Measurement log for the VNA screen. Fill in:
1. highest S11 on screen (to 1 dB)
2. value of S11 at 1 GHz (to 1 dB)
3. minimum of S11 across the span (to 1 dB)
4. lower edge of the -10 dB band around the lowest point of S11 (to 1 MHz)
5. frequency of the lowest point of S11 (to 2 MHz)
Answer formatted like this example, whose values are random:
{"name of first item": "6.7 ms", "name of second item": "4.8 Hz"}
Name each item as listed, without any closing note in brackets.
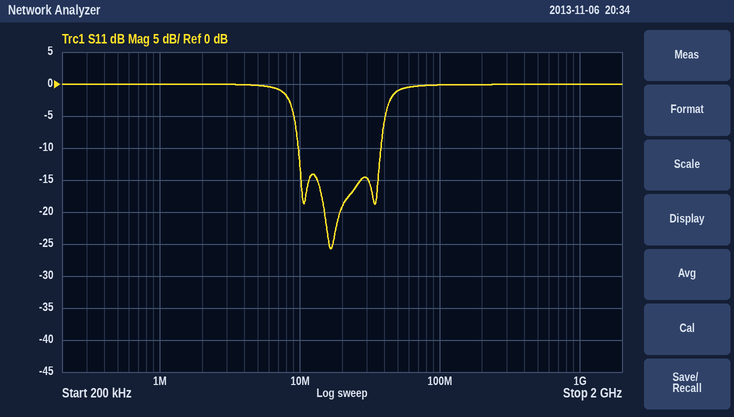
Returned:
{"highest S11 on screen": "0 dB", "value of S11 at 1 GHz": "0 dB", "minimum of S11 across the span": "-26 dB", "lower edge of the -10 dB band around the lowest point of S11": "10 MHz", "frequency of the lowest point of S11": "16 MHz"}
